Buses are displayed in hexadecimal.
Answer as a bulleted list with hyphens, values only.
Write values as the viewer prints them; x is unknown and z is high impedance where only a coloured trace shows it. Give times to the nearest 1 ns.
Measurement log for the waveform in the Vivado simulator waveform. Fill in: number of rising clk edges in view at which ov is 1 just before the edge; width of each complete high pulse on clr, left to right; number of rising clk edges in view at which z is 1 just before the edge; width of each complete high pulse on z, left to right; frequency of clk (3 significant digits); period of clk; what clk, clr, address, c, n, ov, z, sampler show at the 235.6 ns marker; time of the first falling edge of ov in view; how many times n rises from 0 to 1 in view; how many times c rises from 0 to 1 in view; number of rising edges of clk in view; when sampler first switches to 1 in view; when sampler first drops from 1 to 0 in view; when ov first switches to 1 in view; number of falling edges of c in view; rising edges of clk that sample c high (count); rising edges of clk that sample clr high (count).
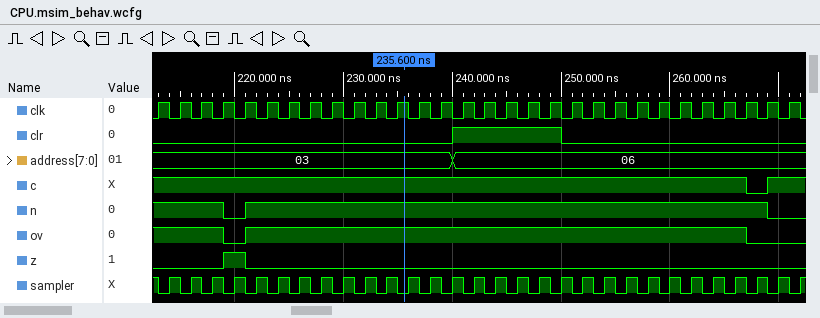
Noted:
- 27
- 10 ns
- 1
- 2 ns
- 500 MHz
- 2 ns
- clk=1, clr=0, address=03, c=1, n=1, ov=1, z=0, sampler=0
- 219 ns
- 1
- 1
- 30
- 214 ns
- 213 ns
- 221 ns
- 1
- 29
- 5
